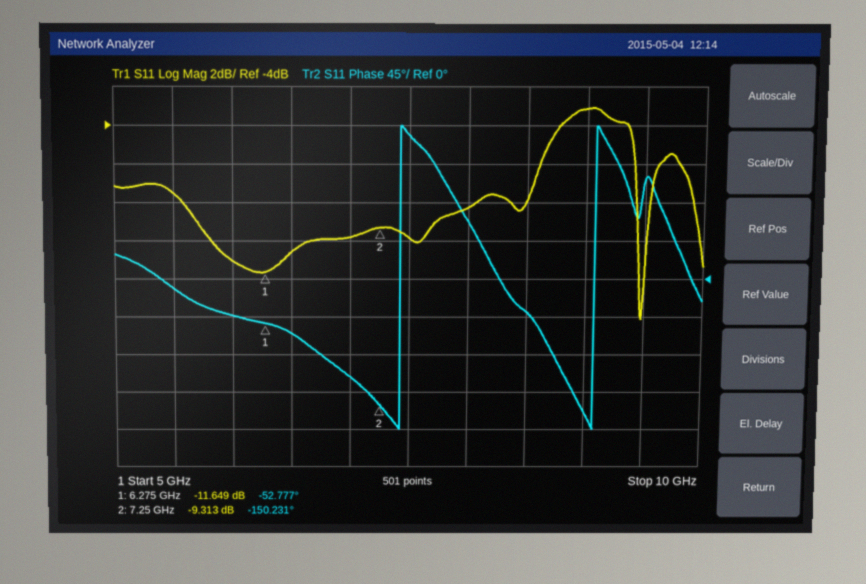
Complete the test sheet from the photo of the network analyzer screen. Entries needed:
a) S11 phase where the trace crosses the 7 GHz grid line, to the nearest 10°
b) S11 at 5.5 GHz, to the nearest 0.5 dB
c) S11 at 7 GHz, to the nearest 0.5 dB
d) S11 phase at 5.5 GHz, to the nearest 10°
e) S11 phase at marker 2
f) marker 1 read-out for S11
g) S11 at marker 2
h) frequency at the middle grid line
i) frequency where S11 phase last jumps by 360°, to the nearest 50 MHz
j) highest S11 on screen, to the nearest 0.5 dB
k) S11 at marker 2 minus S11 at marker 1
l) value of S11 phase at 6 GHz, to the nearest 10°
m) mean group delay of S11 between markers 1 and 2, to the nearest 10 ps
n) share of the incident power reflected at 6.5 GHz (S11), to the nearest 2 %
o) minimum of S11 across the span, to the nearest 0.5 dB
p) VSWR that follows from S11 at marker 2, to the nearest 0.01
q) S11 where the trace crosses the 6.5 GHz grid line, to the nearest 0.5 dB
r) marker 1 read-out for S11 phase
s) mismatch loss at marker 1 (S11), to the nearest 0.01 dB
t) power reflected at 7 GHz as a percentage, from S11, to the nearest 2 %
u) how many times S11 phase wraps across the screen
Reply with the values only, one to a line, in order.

-120°
-7.5 dB
-10.0 dB
-10°
-150.231°
-11.649 dB
-9.313 dB
7.5 GHz
9.10 GHz
-3.0 dB
2.336 dB
-40°
280 ps
8 %
-14.0 dB
2.04
-10.5 dB
-52.777°
0.31 dB
10 %
2
